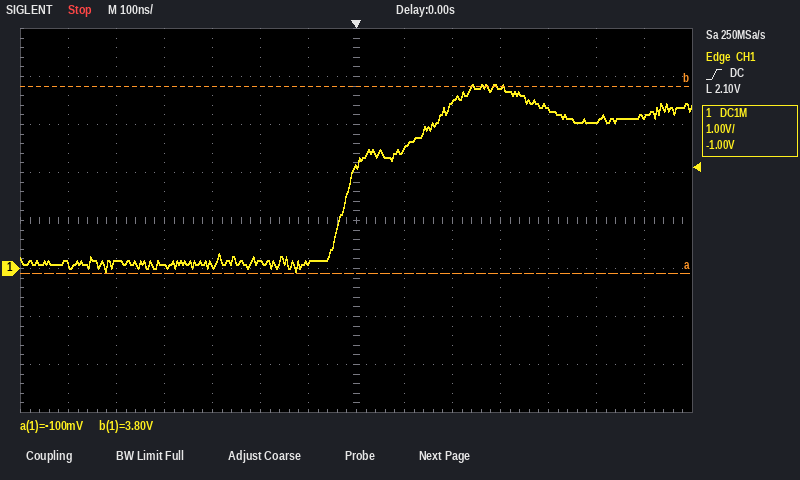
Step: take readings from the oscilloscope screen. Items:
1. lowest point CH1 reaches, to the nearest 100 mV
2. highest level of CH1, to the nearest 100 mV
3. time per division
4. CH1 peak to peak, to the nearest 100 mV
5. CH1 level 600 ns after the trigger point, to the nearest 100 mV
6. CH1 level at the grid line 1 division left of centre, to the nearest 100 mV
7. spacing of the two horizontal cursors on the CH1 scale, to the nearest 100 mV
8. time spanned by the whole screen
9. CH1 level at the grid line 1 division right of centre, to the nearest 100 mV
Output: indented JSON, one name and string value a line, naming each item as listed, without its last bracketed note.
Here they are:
{
  "lowest point CH1 reaches, to the nearest 100 mV": "-100 mV",
  "highest level of CH1, to the nearest 100 mV": "3.8 V",
  "time per division": "100 ns",
  "CH1 peak to peak, to the nearest 100 mV": "3.9 V",
  "CH1 level 600 ns after the trigger point, to the nearest 100 mV": "3.2 V",
  "CH1 level at the grid line 1 division left of centre, to the nearest 100 mV": "100 mV",
  "spacing of the two horizontal cursors on the CH1 scale, to the nearest 100 mV": "3.9 V",
  "time spanned by the whole screen": "1.4 µs",
  "CH1 level at the grid line 1 division right of centre, to the nearest 100 mV": "2.5 V"
}
